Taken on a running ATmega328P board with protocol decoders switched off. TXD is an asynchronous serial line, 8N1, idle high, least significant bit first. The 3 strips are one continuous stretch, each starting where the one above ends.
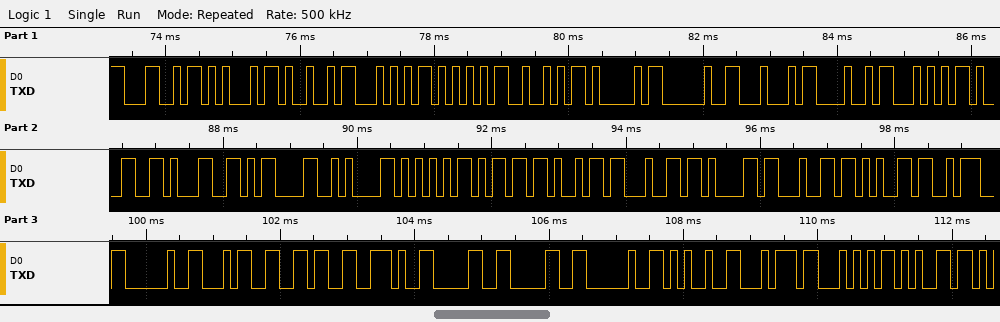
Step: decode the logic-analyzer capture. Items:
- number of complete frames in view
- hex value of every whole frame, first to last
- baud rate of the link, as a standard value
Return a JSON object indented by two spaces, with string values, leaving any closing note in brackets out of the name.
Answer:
{
  "number of complete frames in view": "34",
  "hex value of every whole frame, first to last": "4C 45 49 54 55 52 41 20 44 48 54 31 31 0D 0A 55 6D 69 64 61 64 65 3A 20 34 36 2E 30 30 20 25 74 54 65",
  "baud rate of the link, as a standard value": "9600 baud"
}
